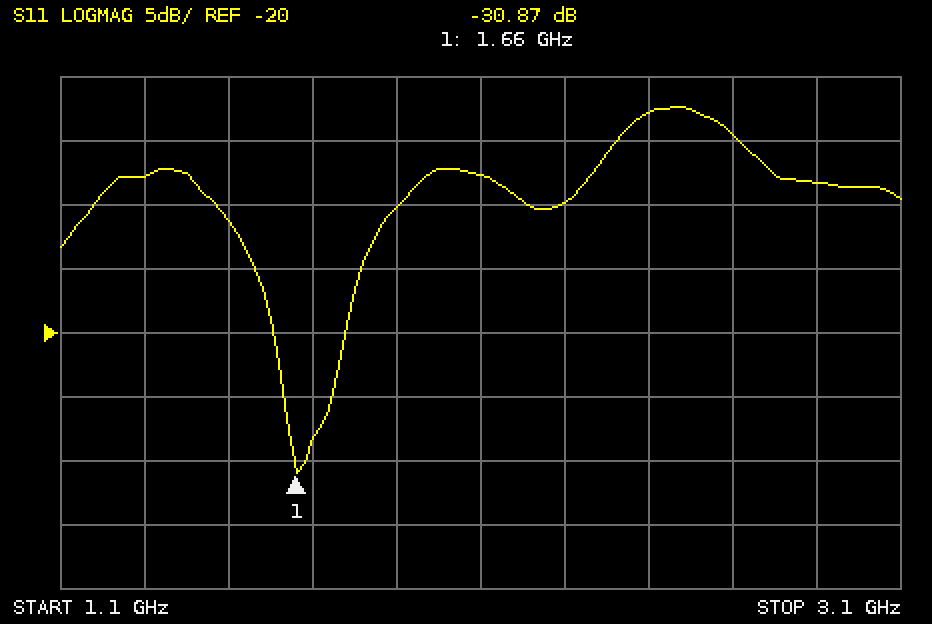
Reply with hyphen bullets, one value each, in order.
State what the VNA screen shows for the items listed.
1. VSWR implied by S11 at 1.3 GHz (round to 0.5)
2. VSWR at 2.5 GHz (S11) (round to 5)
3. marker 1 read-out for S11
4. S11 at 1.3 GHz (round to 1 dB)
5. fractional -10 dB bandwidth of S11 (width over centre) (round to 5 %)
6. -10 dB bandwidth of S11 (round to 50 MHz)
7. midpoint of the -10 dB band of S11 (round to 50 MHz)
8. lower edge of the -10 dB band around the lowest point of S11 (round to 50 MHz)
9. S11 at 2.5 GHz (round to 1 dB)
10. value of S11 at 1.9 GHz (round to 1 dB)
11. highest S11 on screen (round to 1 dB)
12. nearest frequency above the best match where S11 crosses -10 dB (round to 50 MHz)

- 2.5
- 5
- -30.87 dB
- -8 dB
- 25 %
- 450 MHz
- 1.70 GHz
- 1.45 GHz
- -3 dB
- -10 dB
- -2 dB
- 1.90 GHz
